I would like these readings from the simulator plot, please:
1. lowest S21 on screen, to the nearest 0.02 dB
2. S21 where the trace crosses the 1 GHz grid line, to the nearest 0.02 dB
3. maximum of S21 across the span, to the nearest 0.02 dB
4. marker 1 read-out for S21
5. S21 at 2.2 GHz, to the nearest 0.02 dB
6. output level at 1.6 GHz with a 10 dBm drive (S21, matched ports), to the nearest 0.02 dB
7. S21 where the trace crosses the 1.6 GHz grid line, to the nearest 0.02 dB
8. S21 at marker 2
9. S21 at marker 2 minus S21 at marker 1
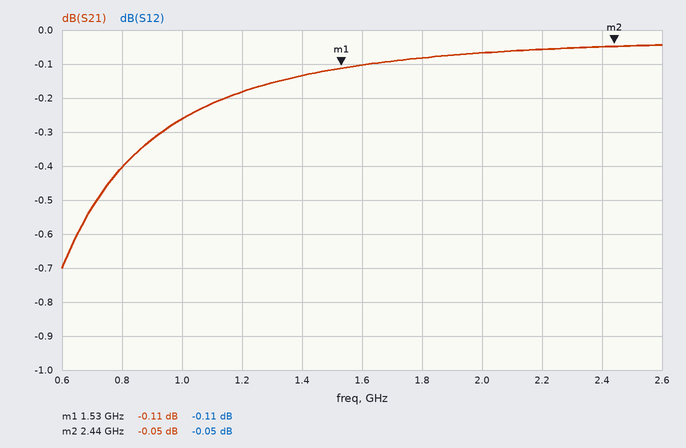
-0.70 dB
-0.26 dB
-0.04 dB
-0.11 dB
-0.06 dB
9.90 dBm
-0.10 dB
-0.05 dB
0.06 dB
